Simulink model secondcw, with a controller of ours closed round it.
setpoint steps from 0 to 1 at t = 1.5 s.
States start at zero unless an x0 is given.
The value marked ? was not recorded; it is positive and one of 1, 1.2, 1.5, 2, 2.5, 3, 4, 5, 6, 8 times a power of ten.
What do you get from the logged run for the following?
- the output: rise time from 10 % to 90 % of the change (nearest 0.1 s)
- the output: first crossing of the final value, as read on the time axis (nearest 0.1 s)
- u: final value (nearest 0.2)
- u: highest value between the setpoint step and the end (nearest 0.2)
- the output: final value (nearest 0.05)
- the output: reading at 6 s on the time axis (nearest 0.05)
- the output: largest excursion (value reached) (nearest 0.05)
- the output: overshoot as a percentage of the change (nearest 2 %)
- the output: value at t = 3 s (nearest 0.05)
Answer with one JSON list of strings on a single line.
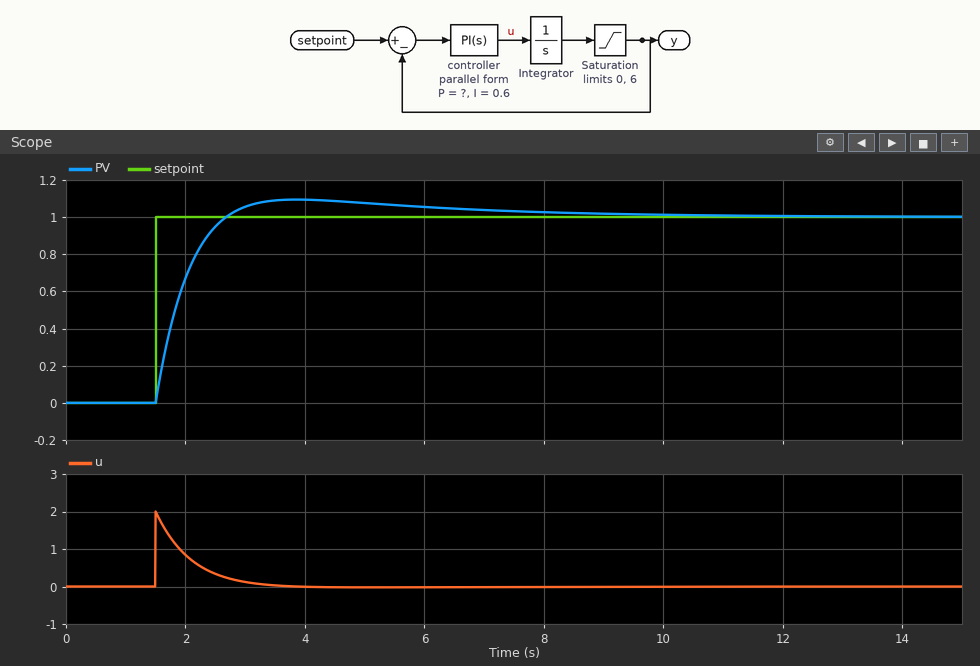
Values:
["0.8 s", "2.7 s", "0.0", "2.0", "1.00", "1.05", "1.10", "10 %", "1.05"]
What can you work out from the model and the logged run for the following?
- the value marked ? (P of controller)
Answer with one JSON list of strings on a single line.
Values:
["2"]
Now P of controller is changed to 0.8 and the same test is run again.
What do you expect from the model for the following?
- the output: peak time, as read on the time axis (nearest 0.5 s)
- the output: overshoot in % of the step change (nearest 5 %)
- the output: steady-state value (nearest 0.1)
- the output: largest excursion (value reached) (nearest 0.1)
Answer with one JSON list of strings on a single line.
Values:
["4.5 s", "30 %", "1.0", "1.3"]
